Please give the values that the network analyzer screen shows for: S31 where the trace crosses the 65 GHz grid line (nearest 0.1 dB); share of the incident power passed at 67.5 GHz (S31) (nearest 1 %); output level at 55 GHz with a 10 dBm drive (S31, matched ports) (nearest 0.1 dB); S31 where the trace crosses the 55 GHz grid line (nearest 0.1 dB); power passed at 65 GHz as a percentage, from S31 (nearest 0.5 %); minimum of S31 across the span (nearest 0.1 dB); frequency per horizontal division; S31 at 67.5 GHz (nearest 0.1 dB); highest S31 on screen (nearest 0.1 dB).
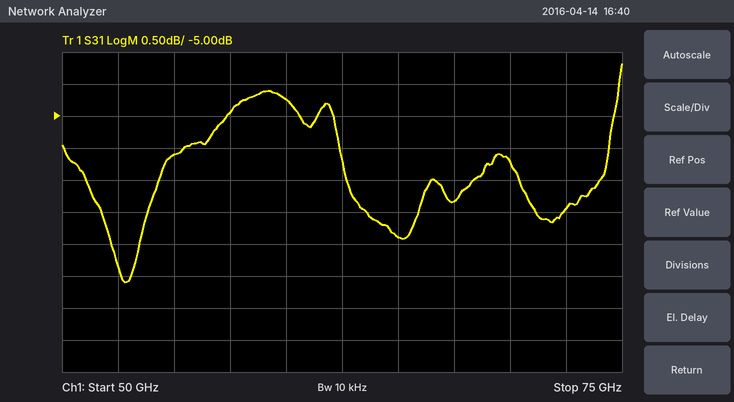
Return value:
-6.9 dB
23 %
4.4 dBm
-5.6 dB
20.5 %
-7.6 dB
2.5 GHz
-6.3 dB
-4.2 dB
